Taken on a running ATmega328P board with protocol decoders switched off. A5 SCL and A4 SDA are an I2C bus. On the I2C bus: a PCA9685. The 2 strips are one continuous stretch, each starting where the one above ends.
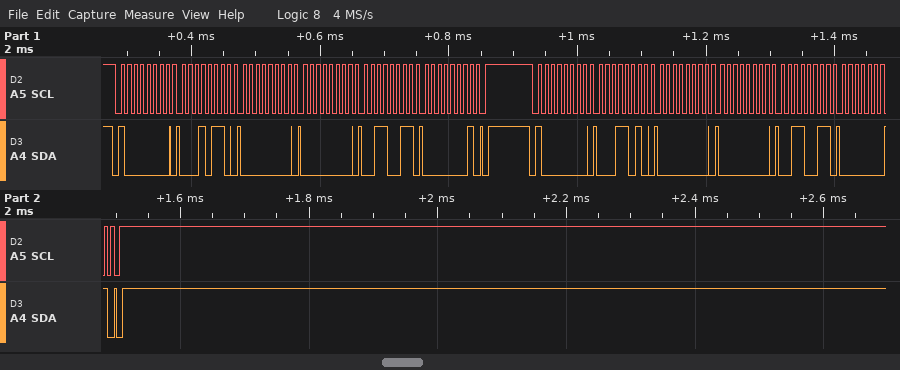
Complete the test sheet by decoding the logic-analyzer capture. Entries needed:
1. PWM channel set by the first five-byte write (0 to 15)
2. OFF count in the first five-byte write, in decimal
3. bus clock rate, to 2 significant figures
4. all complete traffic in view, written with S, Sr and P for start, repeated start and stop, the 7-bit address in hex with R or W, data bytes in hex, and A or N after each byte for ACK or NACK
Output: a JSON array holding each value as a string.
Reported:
["4", "307", "100 kHz", "S 40W A 16 A 00 A 00 A 33 A 01 A P S 40W A 1A A 00 A 00 A 33 A 01 A P"]
